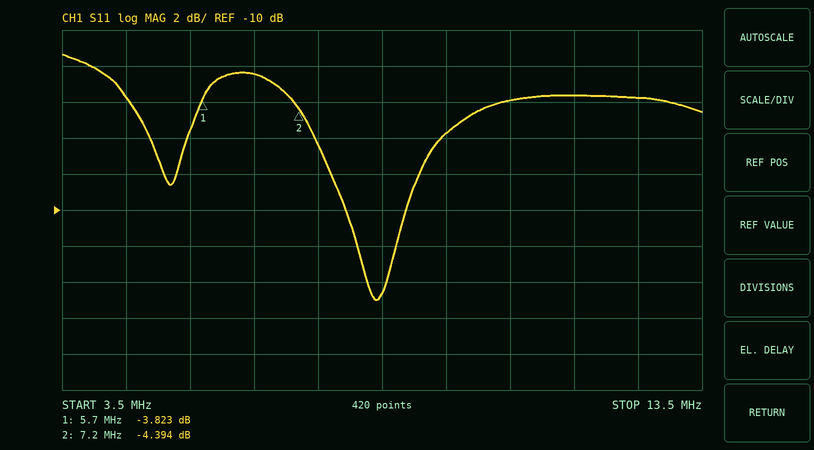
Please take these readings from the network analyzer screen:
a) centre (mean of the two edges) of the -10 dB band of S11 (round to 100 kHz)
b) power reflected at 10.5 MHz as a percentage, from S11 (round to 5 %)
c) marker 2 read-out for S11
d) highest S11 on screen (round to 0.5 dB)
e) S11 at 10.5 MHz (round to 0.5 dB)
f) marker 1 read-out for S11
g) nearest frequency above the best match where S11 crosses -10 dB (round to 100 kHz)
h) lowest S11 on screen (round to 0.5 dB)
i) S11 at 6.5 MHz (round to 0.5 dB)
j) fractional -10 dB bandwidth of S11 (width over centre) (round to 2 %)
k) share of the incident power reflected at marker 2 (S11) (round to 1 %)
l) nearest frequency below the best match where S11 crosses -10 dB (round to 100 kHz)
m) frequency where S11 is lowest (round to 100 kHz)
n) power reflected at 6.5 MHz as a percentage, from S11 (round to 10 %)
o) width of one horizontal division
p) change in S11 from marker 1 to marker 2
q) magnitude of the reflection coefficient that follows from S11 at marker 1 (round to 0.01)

8.4 MHz
40 %
-4.394 dB
-1.5 dB
-4.0 dB
-3.823 dB
8.9 MHz
-15.0 dB
-2.5 dB
12 %
36 %
7.9 MHz
8.4 MHz
60 %
1 MHz
-0.571 dB
0.64
